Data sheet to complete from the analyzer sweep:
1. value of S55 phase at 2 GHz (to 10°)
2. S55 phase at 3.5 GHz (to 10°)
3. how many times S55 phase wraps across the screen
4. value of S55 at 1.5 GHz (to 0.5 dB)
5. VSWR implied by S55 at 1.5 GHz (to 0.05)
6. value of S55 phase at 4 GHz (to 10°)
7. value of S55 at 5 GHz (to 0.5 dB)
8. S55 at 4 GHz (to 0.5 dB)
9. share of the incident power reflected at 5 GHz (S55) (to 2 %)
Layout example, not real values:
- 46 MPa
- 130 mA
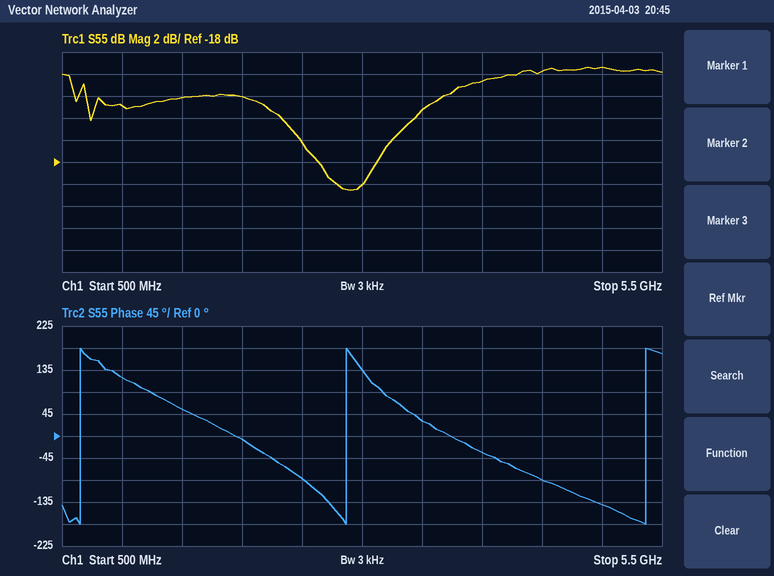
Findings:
- -10°
- 30°
- 3
- -12.0 dB
- 1.65
- -30°
- -9.5 dB
- -10.5 dB
- 12 %
